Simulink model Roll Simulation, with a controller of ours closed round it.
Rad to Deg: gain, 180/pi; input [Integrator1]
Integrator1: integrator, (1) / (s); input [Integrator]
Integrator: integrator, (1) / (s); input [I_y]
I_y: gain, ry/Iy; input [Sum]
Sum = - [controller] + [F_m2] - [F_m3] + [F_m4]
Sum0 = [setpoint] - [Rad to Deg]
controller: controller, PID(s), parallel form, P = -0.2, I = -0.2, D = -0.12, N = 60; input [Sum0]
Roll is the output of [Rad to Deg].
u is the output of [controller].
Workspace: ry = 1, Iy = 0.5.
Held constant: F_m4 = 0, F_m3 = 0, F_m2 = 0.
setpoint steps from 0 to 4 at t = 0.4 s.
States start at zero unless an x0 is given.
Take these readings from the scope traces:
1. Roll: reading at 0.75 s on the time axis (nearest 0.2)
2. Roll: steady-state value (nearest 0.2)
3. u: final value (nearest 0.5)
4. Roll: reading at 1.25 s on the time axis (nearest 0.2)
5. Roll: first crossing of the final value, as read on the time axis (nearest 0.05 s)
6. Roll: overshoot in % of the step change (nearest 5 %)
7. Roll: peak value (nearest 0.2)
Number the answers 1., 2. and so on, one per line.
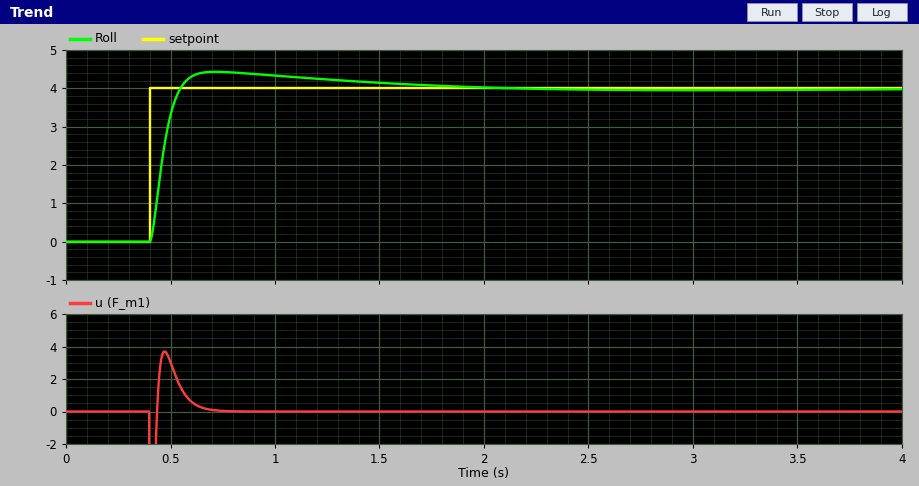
1. 4.4
2. 4.0
3. 0.0
4. 4.2
5. 0.55 s
6. 10 %
7. 4.4
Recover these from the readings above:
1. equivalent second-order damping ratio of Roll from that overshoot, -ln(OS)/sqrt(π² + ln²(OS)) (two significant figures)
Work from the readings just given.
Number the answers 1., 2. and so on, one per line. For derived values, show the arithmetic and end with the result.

1. ln(0.1) = -2.303; 2.303 / sqrt(9.870 + 5.302) = 0.59
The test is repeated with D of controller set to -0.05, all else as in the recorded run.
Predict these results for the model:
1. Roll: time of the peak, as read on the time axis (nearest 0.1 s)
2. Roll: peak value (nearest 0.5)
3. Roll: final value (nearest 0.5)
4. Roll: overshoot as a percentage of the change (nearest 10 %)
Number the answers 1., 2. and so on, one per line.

1. 0.9 s
2. 5.5
3. 4.0
4. 30 %
